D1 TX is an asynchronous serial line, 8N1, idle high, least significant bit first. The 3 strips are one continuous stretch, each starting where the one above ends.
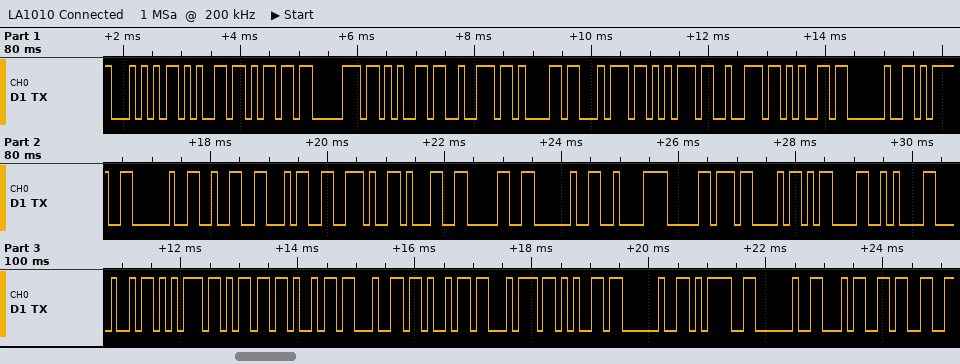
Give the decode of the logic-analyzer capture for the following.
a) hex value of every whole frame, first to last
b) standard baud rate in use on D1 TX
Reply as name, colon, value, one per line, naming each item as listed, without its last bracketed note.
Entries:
hex value of every whole frame, first to last: 54 65 6D 70 65 72 61 74 75 72 65 20 3D 20 32 34 2E 31 30 20 C2 B0 43 0D 0A 48 75 6D 69 64 69 74 65 20 3D 20 34 33
standard baud rate in use on D1 TX: 9600 baud
